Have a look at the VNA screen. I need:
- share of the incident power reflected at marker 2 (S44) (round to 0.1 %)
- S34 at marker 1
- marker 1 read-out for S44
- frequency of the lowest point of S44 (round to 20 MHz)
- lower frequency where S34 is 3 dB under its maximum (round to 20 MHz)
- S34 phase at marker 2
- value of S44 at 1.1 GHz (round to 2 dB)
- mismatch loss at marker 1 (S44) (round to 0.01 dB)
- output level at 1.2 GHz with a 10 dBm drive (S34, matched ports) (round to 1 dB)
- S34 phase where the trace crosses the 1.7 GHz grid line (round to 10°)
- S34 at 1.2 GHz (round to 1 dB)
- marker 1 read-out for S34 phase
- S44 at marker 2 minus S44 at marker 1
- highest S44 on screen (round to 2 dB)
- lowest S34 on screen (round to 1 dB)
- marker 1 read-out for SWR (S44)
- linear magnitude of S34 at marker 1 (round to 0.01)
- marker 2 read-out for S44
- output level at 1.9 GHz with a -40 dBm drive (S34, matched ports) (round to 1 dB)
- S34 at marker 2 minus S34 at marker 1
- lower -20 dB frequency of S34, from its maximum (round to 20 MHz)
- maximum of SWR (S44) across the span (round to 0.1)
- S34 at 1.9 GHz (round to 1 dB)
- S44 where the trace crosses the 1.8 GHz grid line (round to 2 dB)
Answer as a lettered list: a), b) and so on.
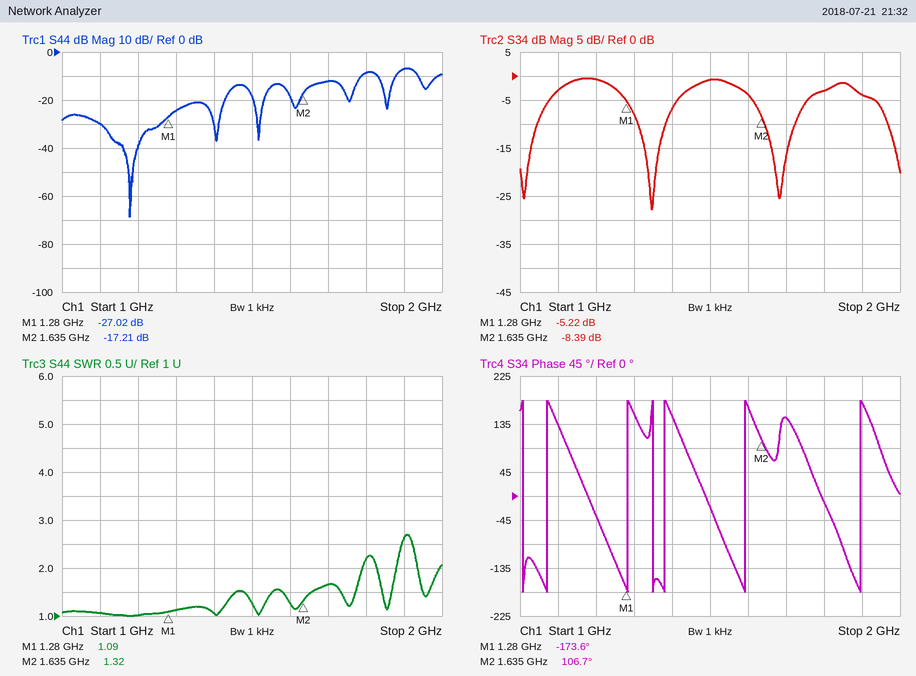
a) 1.9 %
b) -5.22 dB
c) -27.02 dB
d) 1.18 GHz
e) 1.10 GHz
f) 106.7°
g) -30 dB
h) 0.01 dB
i) 9 dBm
j) 150°
k) -1 dB
l) -173.6°
m) 9.81 dB
n) -6 dB
o) -28 dB
p) 1.09
q) 0.55
r) -17.21 dB
s) -44 dBm
t) -3.17 dB
u) 1.02 GHz
v) 2.7
w) -4 dB
x) -8 dB
